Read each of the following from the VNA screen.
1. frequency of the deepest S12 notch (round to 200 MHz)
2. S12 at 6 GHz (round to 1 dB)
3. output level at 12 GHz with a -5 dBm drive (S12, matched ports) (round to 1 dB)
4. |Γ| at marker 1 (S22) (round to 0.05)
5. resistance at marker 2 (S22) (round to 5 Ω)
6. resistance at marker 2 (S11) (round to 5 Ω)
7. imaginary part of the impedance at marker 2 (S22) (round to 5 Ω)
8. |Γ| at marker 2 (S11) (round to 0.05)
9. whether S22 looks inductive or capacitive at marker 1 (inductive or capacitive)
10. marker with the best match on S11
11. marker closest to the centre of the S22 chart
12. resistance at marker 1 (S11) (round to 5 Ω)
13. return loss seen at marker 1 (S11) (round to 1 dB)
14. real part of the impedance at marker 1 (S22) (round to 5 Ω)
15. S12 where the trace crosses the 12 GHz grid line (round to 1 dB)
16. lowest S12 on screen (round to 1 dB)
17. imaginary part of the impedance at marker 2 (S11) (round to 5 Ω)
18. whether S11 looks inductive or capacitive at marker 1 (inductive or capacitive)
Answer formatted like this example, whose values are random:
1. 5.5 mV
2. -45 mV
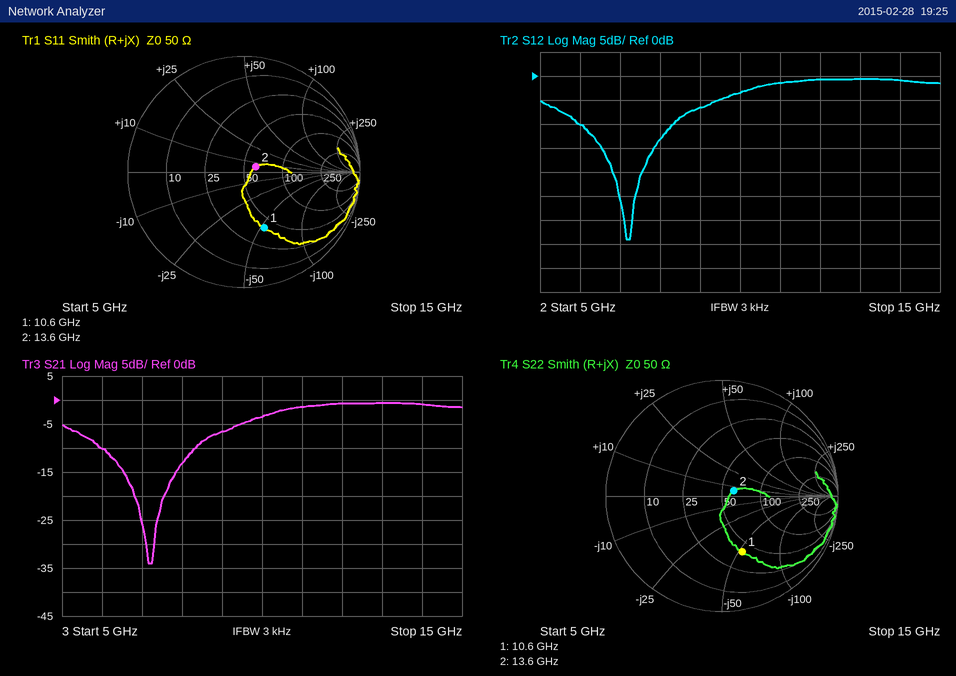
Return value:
1. 7.2 GHz
2. -10 dB
3. -6 dBm
4. 0.50
5. 60 Ω
6. 60 Ω
7. +5 Ω
8. 0.10
9. capacitive
10. marker 2
11. marker 2
12. 40 Ω
13. 6 dB
14. 40 Ω
15. -1 dB
16. -34 dB
17. +5 Ω
18. capacitive
